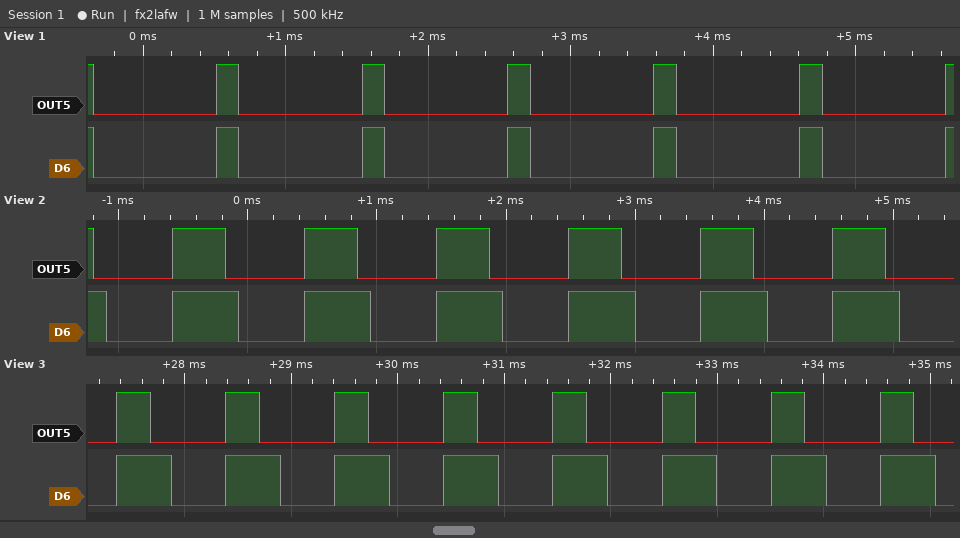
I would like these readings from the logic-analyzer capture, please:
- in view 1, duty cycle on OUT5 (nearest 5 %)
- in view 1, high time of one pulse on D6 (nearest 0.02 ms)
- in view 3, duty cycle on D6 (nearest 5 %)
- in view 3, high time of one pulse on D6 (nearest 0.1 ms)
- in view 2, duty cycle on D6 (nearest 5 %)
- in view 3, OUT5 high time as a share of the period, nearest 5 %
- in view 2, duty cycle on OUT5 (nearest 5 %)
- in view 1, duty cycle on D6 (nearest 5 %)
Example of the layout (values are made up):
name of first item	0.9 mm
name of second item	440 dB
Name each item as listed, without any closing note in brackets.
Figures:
in view 1, duty cycle on OUT5	15 %
in view 1, high time of one pulse on D6	0.16 ms
in view 3, duty cycle on D6	50 %
in view 3, high time of one pulse on D6	0.5 ms
in view 2, duty cycle on D6	50 %
in view 3, OUT5 high time as a share of the period, nearest 5 %	30 %
in view 2, duty cycle on OUT5	40 %
in view 1, duty cycle on D6	15 %
